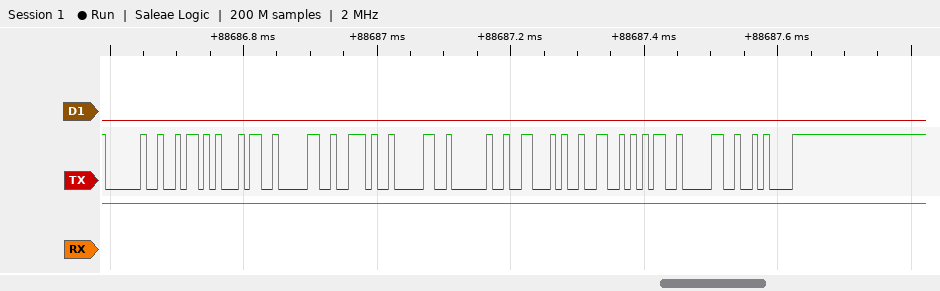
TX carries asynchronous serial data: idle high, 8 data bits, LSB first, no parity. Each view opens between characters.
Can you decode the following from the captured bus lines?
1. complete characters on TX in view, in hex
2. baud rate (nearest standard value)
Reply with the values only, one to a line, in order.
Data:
20, 5A, 34, 30, 2E, 30, 20, 46, 32, 35, 30, 0A
115200 baud
